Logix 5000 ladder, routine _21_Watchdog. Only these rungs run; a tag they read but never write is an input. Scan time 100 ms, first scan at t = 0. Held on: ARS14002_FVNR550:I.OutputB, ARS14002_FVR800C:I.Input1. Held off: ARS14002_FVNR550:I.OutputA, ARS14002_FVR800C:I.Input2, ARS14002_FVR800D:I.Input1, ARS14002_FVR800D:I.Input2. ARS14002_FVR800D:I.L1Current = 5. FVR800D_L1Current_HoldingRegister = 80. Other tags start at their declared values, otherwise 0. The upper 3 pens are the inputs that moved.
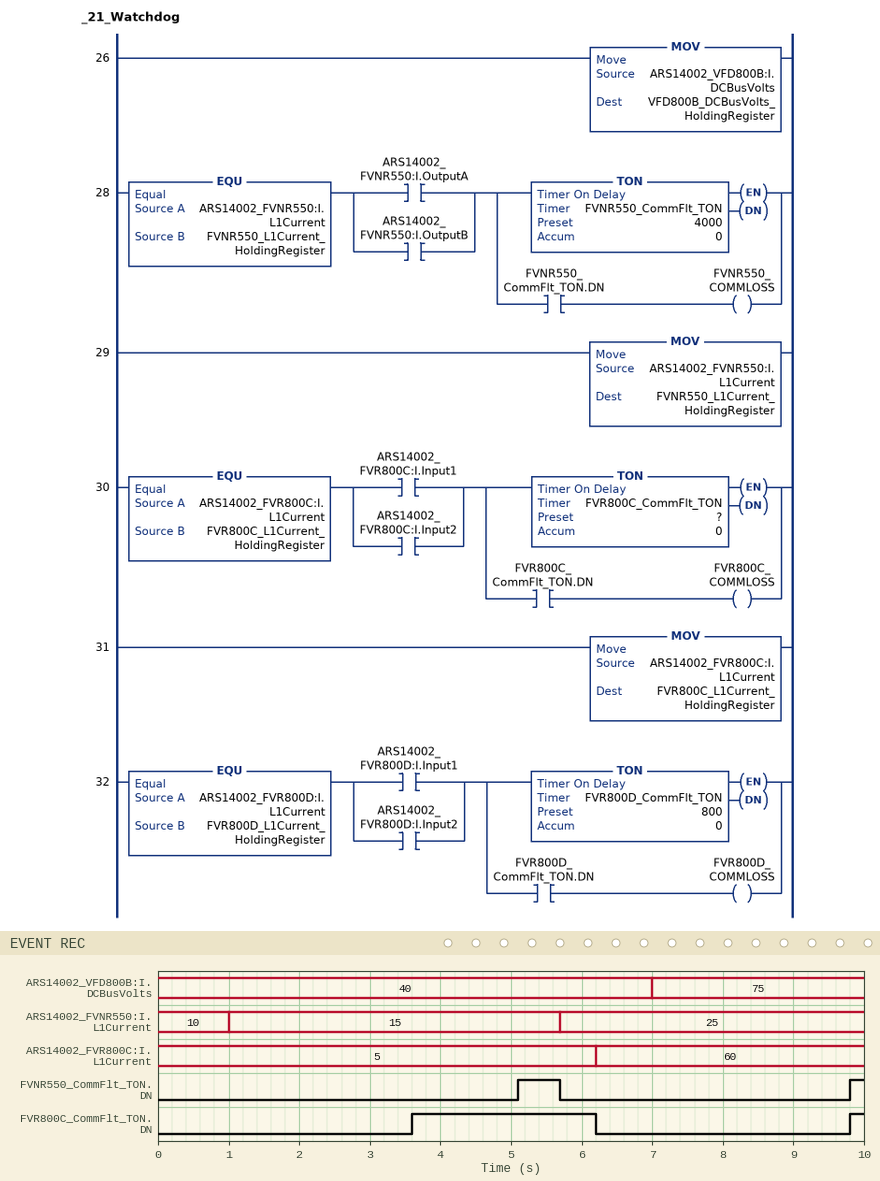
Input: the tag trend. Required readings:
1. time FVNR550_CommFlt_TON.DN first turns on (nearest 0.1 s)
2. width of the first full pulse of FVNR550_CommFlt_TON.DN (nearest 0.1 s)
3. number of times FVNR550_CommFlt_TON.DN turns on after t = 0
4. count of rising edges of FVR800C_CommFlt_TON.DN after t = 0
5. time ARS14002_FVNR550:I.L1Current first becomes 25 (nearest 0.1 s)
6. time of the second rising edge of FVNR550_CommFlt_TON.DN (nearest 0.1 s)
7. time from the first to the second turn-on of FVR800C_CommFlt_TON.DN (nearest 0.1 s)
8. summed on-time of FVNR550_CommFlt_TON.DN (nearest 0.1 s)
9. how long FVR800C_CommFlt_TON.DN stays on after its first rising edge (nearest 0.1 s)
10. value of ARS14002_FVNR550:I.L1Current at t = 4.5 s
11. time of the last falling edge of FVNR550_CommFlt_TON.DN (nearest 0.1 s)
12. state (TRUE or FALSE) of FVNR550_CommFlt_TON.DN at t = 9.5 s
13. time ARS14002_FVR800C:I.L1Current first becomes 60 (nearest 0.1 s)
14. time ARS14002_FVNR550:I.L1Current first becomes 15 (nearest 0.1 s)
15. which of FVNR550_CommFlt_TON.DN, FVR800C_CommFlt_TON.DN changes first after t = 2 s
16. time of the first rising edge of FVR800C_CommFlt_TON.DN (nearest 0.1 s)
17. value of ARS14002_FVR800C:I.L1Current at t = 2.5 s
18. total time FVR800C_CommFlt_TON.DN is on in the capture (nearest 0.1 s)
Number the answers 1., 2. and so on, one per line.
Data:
1. 5.1 s
2. 0.6 s
3. 2
4. 2
5. 5.7 s
6. 9.8 s
7. 6.2 s
8. 0.8 s
9. 2.6 s
10. 15
11. 5.7 s
12. FALSE
13. 6.2 s
14. 1.0 s
15. FVR800C_CommFlt_TON.DN
16. 3.6 s
17. 5
18. 2.8 s
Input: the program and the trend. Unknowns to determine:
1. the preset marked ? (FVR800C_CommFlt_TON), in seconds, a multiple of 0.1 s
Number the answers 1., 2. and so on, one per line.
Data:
1. 3.5 s
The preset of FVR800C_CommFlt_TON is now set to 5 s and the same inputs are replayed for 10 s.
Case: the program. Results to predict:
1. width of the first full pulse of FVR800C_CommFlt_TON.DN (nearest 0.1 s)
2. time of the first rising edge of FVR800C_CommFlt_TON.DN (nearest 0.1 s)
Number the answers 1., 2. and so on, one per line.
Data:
1. 1.1 s
2. 5.1 s
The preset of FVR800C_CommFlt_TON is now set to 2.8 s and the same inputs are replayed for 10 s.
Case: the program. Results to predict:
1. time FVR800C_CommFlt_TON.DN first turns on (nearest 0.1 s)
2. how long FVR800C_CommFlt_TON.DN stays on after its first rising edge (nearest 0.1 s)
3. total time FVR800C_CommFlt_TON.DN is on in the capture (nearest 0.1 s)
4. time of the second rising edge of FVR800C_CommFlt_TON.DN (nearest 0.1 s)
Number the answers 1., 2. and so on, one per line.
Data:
1. 2.9 s
2. 3.3 s
3. 4.2 s
4. 9.1 s
